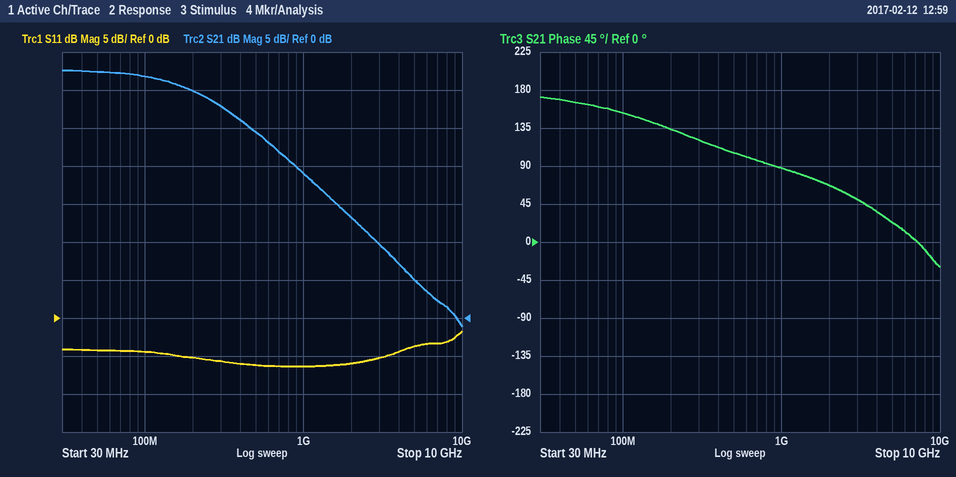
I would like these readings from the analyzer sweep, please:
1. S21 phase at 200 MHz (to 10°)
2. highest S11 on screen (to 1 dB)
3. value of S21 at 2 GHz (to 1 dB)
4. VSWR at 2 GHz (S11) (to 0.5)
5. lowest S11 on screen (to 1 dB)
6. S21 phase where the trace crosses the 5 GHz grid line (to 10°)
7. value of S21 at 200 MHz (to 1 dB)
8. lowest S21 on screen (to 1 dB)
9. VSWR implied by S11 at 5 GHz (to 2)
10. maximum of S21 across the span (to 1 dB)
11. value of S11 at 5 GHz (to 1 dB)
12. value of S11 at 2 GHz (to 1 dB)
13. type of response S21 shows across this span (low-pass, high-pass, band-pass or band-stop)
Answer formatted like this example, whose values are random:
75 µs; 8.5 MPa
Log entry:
130°; -2 dB; 13 dB; 3.0; -6 dB; 20°; 30 dB; -1 dB; 4; 33 dB; -4 dB; -6 dB; low-pass
